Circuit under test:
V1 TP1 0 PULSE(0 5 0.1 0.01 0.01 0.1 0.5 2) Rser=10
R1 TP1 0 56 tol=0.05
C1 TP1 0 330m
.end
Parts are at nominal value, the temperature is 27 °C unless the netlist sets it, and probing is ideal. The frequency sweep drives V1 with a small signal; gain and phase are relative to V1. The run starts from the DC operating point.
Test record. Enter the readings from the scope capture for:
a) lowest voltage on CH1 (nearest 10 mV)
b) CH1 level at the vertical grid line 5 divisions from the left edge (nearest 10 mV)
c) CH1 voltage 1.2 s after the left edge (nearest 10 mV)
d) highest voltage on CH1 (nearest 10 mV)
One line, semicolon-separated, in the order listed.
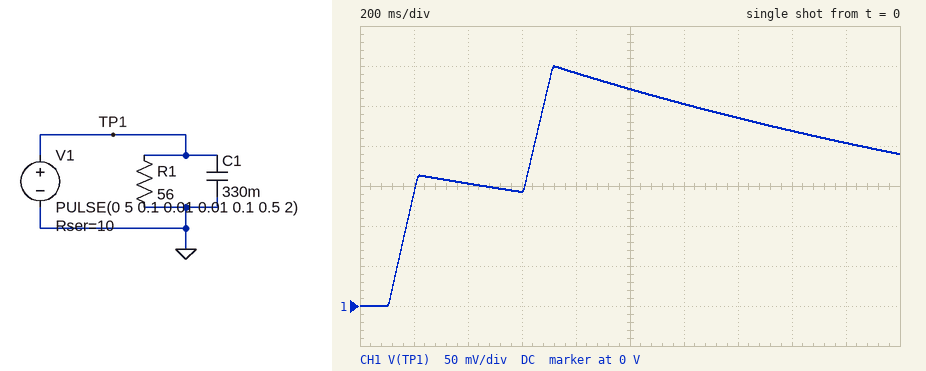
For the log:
0 V; 270 mV; 250 mV; 300 mV
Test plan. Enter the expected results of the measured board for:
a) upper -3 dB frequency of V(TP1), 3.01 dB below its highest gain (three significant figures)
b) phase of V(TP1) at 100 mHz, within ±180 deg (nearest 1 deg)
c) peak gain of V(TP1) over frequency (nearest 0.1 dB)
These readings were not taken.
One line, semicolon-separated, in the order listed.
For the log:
56.8 mHz; -60 deg; -1.4 dB
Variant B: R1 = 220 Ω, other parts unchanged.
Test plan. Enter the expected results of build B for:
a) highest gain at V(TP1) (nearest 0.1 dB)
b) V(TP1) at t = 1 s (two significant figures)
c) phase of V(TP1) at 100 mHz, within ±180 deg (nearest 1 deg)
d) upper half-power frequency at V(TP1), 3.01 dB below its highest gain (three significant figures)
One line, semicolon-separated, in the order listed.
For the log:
-0.4 dB; 280 mV; -63 deg; 50.4 mHz
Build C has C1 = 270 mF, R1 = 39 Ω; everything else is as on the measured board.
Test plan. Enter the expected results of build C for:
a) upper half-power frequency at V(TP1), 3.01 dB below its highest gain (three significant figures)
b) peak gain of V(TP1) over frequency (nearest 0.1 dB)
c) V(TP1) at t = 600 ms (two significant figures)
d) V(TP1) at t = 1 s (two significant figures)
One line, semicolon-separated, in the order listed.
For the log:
74.1 mHz; -2.0 dB; 170 mV; 310 mV
